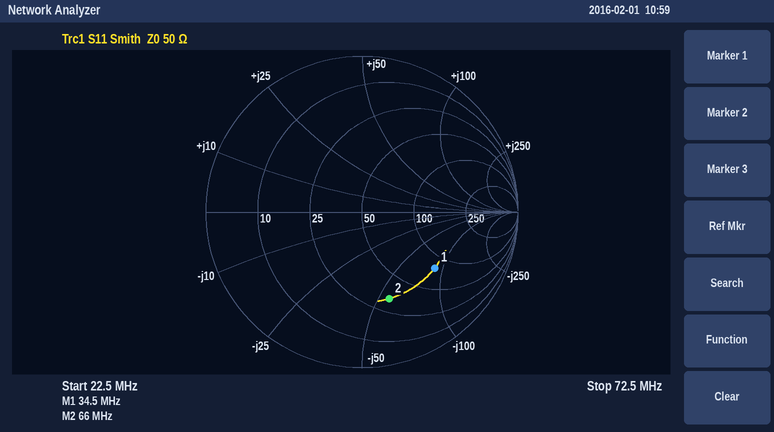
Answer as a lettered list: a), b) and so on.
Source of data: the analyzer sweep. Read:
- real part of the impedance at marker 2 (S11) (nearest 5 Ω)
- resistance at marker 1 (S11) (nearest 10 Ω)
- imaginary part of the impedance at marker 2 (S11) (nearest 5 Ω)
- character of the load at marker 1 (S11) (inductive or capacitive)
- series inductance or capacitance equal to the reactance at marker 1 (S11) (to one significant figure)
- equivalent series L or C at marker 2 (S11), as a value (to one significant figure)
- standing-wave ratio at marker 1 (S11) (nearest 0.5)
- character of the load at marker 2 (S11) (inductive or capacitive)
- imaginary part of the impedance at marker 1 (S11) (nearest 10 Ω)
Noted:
a) 35 Ω
b) 80 Ω
c) -55 Ω
d) capacitive
e) 50 pF
f) 40 pF
g) 4.0
h) capacitive
i) -90 Ω
